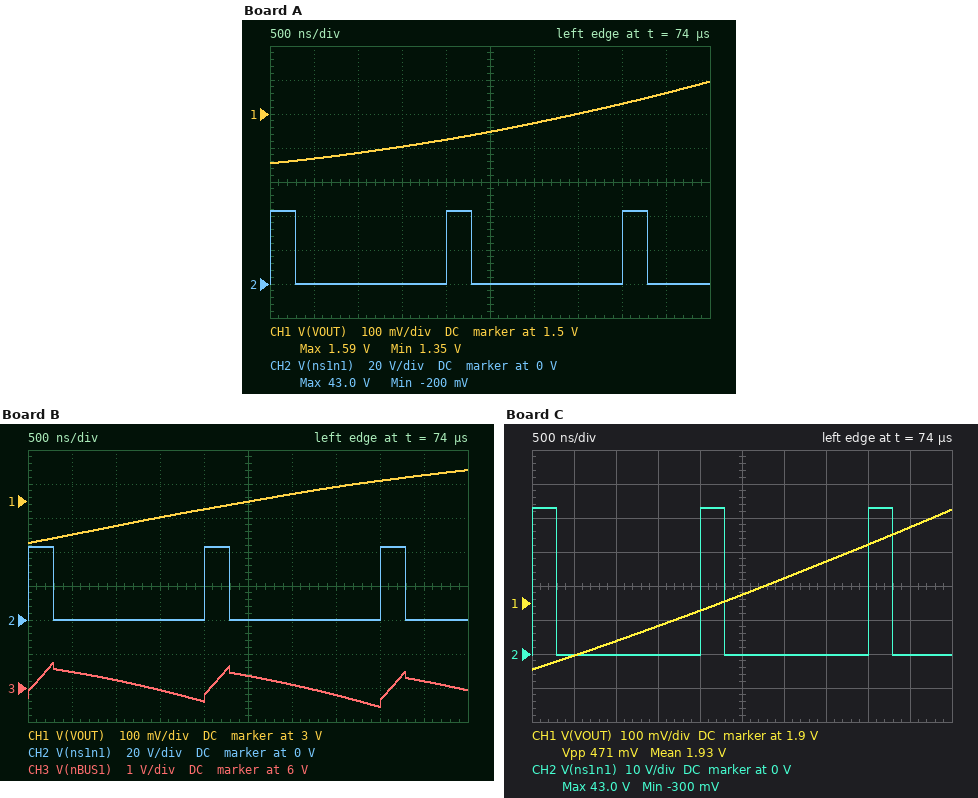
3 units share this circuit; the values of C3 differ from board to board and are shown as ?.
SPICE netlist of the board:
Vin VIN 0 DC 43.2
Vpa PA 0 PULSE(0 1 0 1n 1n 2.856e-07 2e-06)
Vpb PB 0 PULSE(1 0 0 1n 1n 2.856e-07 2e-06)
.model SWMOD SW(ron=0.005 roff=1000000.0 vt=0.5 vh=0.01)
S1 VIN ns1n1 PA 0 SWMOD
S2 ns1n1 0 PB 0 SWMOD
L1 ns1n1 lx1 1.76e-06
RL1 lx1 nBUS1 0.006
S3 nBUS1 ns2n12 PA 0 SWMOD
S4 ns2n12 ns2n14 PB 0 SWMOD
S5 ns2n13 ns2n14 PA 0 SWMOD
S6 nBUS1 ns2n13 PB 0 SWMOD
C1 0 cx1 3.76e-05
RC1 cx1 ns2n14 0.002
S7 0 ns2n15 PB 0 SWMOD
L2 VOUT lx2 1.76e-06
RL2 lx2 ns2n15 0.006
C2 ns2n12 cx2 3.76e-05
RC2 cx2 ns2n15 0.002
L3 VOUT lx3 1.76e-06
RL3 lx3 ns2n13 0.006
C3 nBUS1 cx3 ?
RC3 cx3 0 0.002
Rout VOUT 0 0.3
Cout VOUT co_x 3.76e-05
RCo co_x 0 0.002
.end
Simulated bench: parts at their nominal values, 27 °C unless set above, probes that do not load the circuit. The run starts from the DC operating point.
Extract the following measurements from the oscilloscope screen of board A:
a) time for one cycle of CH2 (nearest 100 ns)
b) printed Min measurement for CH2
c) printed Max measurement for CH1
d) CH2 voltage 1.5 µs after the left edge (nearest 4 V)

2.0 µs
-200 mV
1.59 V
0 V
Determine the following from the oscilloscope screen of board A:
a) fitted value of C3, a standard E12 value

82 µF
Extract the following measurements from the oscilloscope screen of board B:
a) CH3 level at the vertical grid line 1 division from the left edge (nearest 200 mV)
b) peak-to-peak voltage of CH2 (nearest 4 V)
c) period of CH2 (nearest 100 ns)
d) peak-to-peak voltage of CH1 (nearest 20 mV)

6.4 V
44 V
2.0 µs
220 mV
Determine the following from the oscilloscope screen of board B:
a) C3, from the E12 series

27 µF
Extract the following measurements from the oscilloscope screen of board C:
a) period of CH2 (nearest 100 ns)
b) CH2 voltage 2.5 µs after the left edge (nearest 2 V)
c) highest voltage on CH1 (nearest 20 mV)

2.0 µs
0 V
2.18 V
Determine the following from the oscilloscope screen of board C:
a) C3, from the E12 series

68 µF
